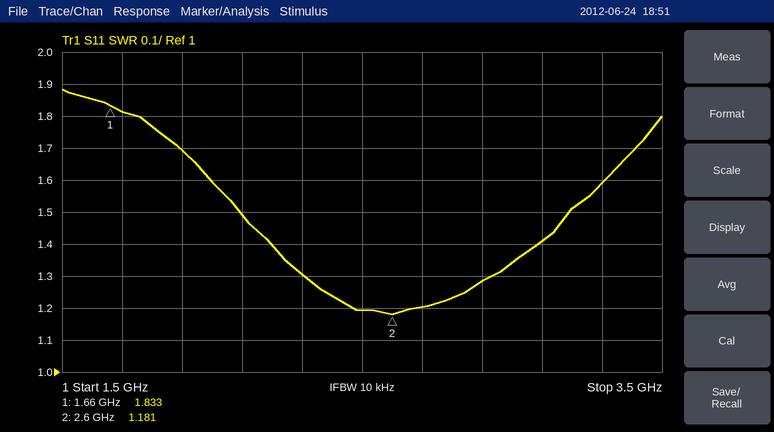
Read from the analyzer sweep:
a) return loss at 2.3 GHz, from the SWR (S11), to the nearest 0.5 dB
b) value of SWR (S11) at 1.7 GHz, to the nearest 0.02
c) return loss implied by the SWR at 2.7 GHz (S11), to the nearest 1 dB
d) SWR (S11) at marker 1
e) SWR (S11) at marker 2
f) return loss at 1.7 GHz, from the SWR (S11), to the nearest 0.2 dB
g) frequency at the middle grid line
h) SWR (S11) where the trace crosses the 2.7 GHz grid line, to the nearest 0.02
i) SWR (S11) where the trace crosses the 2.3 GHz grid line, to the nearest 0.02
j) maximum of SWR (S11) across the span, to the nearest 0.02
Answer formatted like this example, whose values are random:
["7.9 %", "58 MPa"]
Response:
["17.5 dB", "1.82", "21 dB", "1.833", "1.181", "10.8 dB", "2.5 GHz", "1.20", "1.30", "1.88"]
